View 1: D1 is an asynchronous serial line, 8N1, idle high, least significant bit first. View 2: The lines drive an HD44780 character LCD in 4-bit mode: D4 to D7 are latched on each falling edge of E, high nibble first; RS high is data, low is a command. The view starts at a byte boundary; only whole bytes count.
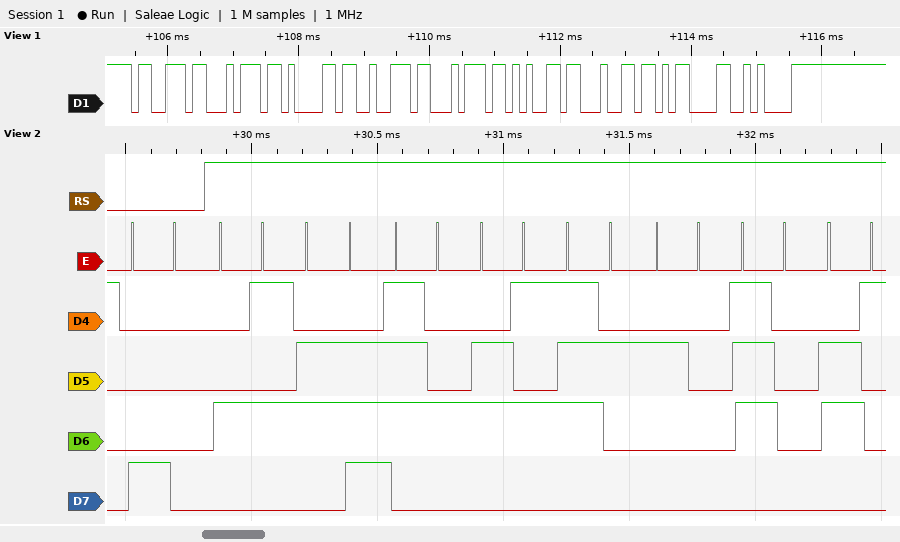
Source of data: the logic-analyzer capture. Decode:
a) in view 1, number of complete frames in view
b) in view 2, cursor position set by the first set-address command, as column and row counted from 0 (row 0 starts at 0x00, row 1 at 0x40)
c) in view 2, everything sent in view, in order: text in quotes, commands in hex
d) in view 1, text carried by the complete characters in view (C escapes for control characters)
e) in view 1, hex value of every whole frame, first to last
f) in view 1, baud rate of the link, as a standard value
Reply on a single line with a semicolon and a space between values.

9; column 0, row 0; 0x80 "Enter pa"; "started\r\n"; 73 74 61 72 74 65 64 0D 0A; 9600 baud
